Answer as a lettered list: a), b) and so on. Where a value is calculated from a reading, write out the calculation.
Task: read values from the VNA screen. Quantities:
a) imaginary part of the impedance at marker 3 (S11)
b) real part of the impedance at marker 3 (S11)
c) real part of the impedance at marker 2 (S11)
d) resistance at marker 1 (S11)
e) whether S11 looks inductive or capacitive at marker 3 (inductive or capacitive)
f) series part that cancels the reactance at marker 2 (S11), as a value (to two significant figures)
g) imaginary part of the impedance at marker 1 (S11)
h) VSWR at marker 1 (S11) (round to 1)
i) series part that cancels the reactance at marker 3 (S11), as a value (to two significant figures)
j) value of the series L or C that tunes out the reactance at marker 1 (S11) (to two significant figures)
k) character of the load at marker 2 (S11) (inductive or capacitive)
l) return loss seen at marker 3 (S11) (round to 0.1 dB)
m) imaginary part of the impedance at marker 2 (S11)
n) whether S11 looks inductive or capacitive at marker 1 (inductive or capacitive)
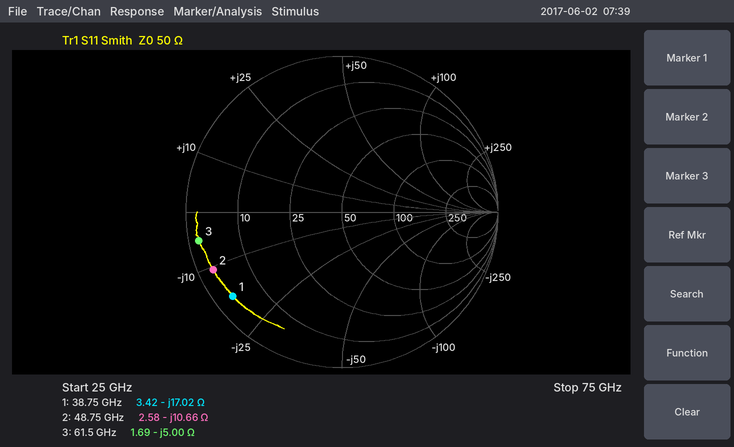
a) -5.00 Ω
b) 1.69 Ω
c) 2.58 Ω
d) 3.42 Ω
e) capacitive
f) L = 10.66 Ω/(2π × 48.75 GHz) ≈ 35 pH
g) -17.02 Ω
h) 16
i) L = 5 Ω/(2π × 61.5 GHz) ≈ 13 pH
j) L = 17.02 Ω/(2π × 38.75 GHz) ≈ 70 pH
k) capacitive
l) 0.6 dB
m) -10.66 Ω
n) capacitive
